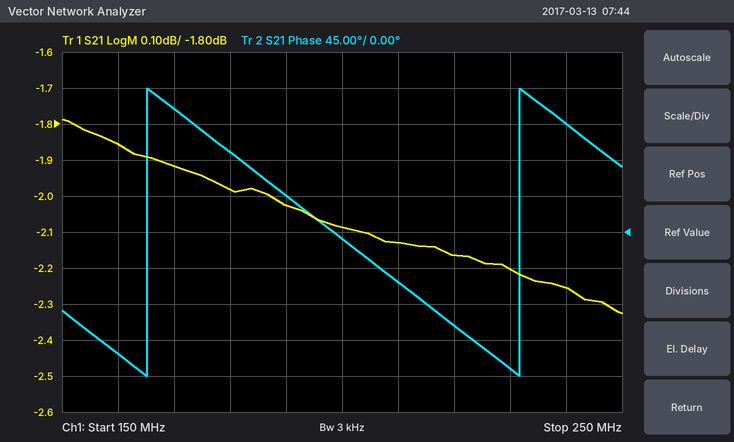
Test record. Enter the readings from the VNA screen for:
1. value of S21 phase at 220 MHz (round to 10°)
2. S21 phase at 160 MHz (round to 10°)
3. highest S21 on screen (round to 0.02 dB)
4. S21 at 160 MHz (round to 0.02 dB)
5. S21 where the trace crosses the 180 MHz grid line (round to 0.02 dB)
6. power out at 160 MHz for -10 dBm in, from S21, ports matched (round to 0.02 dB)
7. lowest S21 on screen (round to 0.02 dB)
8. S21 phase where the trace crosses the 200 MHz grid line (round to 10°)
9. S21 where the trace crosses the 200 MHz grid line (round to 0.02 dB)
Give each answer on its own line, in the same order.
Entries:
-120°
-150°
-1.78 dB
-1.86 dB
-1.98 dB
-11.86 dBm
-2.32 dB
-10°
-2.08 dB
